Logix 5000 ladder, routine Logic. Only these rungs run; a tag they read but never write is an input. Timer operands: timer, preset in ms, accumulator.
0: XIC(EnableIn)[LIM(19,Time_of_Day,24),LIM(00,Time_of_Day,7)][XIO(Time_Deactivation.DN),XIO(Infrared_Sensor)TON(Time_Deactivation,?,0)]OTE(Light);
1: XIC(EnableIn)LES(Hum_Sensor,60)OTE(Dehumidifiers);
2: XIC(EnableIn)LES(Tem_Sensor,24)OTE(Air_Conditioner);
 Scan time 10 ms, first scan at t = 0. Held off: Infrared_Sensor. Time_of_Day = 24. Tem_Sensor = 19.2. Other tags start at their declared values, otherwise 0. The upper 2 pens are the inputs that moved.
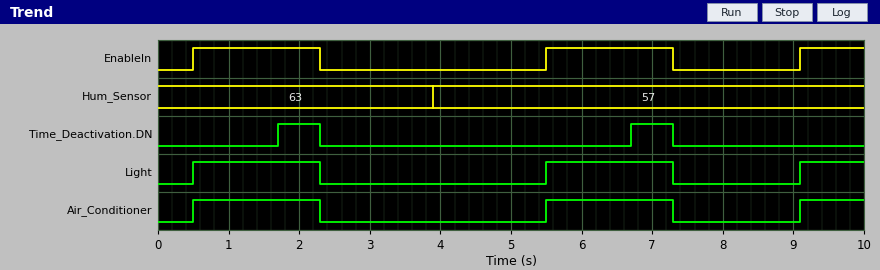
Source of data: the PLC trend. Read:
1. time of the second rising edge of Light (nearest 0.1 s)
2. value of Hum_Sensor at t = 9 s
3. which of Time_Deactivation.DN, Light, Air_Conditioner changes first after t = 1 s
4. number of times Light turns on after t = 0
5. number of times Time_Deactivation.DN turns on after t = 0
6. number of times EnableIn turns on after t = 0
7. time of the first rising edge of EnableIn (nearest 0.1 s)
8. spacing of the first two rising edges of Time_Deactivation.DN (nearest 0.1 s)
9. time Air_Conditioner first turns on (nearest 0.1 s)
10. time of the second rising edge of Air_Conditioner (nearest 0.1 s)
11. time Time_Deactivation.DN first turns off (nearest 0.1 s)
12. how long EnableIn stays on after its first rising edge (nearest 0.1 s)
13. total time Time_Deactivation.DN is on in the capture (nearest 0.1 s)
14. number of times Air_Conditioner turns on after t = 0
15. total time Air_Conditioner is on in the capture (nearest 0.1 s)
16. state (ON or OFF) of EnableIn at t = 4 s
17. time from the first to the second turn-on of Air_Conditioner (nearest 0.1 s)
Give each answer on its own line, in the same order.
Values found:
5.5 s
57
Time_Deactivation.DN
3
2
3
0.5 s
5.0 s
0.5 s
5.5 s
2.3 s
1.8 s
1.2 s
3
4.5 s
OFF
5.0 s
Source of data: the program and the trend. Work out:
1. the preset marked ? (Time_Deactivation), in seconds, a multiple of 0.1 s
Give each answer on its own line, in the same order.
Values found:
1.2 s
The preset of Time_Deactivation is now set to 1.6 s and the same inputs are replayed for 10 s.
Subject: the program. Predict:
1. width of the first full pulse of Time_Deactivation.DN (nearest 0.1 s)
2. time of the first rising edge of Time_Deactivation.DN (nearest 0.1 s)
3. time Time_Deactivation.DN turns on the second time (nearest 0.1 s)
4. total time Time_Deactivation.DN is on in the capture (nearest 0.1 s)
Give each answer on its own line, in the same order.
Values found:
0.2 s
2.1 s
7.1 s
0.4 s
